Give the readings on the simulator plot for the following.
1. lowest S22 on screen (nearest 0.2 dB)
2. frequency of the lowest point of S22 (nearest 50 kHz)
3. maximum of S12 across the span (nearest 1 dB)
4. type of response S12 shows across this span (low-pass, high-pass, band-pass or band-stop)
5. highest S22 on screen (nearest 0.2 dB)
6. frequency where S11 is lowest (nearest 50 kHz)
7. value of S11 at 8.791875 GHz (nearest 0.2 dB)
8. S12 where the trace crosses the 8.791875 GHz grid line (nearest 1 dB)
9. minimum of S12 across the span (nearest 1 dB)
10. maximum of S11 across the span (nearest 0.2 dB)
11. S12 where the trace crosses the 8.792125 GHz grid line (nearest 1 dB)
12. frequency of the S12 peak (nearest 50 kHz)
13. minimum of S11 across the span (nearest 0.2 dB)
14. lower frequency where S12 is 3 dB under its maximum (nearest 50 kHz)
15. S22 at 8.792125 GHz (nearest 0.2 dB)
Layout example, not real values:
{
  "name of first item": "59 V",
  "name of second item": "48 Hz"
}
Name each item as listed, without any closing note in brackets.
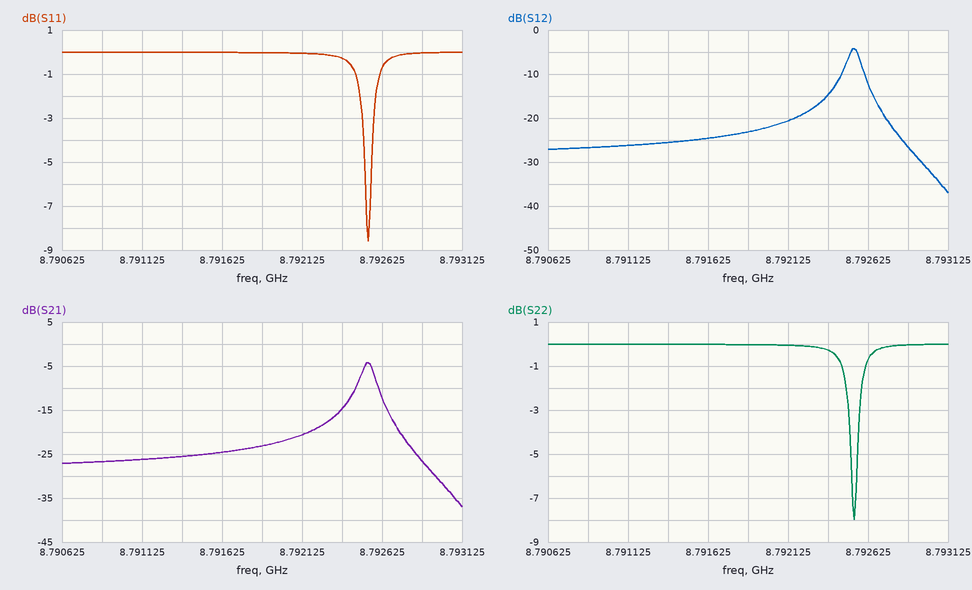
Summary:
{
  "lowest S22 on screen": "-8.0 dB",
  "frequency of the lowest point of S22": "8.79255 GHz",
  "maximum of S12 across the span": "-4 dB",
  "type of response S12 shows across this span": "band-pass",
  "highest S22 on screen": "0.0 dB",
  "frequency where S11 is lowest": "8.79255 GHz",
  "value of S11 at 8.791875 GHz": "0.0 dB",
  "S12 where the trace crosses the 8.791875 GHz grid line": "-23 dB",
  "minimum of S12 across the span": "-37 dB",
  "maximum of S11 across the span": "0.0 dB",
  "S12 where the trace crosses the 8.792125 GHz grid line": "-21 dB",
  "frequency of the S12 peak": "8.79255 GHz",
  "minimum of S11 across the span": "-8.6 dB",
  "lower frequency where S12 is 3 dB under its maximum": "8.79250 GHz",
  "S22 at 8.792125 GHz": "0.0 dB"
}
